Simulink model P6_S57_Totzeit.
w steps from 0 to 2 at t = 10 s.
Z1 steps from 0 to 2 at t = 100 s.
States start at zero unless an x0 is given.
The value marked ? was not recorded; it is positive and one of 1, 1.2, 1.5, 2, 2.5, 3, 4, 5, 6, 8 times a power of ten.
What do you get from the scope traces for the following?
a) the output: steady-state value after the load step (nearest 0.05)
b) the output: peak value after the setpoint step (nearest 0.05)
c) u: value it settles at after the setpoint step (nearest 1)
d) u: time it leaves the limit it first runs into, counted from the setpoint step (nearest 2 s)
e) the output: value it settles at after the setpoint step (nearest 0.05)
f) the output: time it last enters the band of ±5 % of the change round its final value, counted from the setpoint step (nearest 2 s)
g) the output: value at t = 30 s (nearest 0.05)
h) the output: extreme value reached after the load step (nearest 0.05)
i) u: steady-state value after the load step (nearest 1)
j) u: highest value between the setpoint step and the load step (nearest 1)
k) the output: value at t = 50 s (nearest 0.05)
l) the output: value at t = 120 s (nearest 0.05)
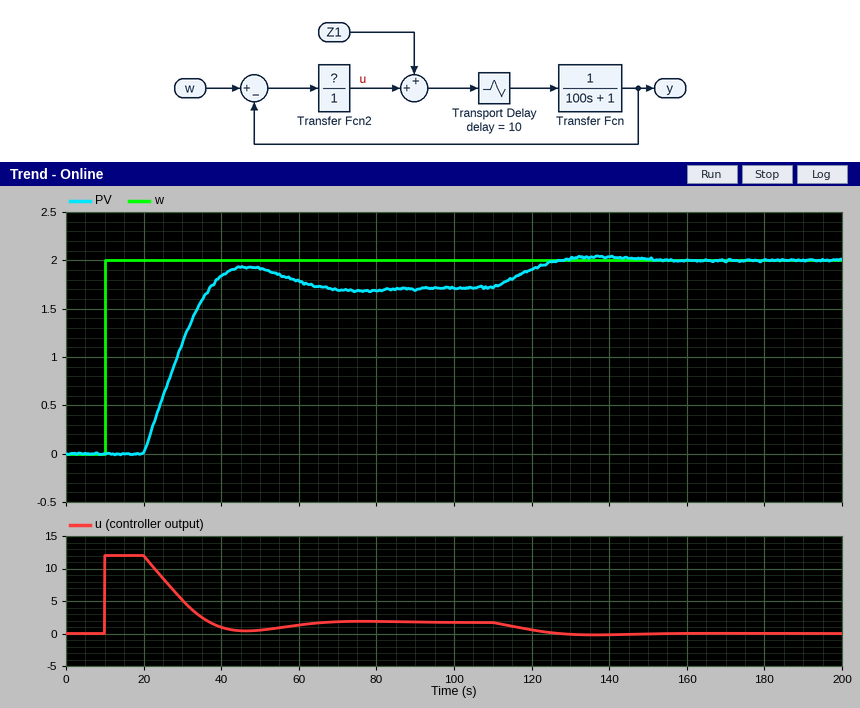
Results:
2.00
1.95
2
10 s
1.70
48 s
1.15
2.05
0
12
1.90
1.90
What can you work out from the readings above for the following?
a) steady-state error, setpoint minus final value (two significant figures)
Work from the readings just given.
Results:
0.30
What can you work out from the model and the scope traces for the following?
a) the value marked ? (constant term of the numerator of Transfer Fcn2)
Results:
6
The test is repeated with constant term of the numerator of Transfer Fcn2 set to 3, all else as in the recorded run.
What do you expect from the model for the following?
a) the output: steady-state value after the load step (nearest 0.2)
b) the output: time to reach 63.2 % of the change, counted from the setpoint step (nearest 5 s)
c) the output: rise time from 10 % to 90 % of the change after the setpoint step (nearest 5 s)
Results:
2.0
30 s
35 s
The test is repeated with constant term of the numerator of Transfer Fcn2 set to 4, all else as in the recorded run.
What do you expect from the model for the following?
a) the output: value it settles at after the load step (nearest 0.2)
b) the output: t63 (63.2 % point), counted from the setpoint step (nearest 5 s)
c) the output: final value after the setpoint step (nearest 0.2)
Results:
2.0
25 s
1.6
